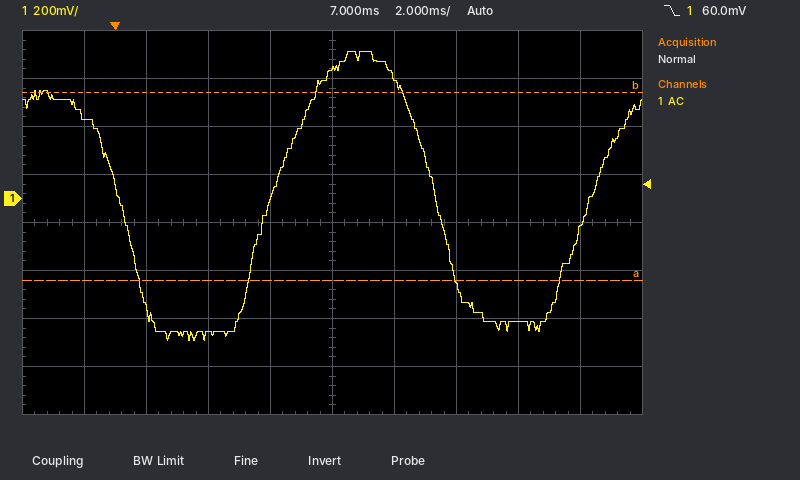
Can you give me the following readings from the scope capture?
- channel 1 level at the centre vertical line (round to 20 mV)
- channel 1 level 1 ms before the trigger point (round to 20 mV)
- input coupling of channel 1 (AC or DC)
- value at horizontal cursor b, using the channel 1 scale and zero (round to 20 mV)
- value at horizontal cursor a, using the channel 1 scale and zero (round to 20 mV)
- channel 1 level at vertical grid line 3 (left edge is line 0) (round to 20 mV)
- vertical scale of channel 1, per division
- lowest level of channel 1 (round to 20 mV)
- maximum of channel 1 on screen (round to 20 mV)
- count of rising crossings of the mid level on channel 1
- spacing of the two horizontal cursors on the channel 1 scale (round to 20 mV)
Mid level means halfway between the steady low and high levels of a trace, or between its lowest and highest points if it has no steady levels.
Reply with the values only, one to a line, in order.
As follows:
540 mV
340 mV
AC
440 mV
-340 mV
-560 mV
200 mV
-600 mV
620 mV
2
780 mV
